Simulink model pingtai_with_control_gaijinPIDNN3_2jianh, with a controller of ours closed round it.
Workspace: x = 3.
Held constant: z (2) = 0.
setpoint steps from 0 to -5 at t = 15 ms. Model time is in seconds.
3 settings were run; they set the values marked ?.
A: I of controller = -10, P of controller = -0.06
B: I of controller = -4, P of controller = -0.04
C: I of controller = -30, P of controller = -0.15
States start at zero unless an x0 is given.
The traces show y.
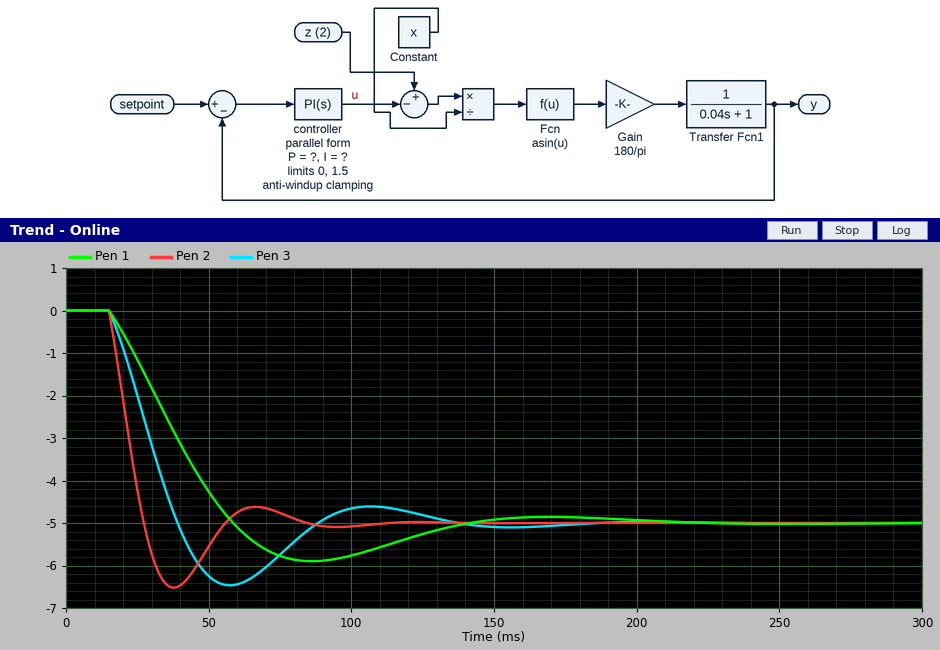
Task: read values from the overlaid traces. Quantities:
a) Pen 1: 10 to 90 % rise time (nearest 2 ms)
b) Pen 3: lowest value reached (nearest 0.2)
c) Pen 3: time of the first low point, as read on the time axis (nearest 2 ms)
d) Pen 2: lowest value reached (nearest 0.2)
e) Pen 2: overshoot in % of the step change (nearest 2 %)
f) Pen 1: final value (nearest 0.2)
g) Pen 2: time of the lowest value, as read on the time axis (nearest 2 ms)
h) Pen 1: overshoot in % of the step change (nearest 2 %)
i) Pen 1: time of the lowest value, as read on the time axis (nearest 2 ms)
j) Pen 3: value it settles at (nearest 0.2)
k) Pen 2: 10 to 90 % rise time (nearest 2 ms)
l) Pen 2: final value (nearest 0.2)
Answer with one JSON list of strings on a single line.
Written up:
["32 ms", "-6.4", "58 ms", "-6.6", "30 %", "-5.0", "38 ms", "18 %", "86 ms", "-5.0", "10 ms", "-5.0"]
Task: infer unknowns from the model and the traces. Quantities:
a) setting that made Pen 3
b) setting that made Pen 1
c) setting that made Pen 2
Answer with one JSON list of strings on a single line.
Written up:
["A", "B", "C"]
